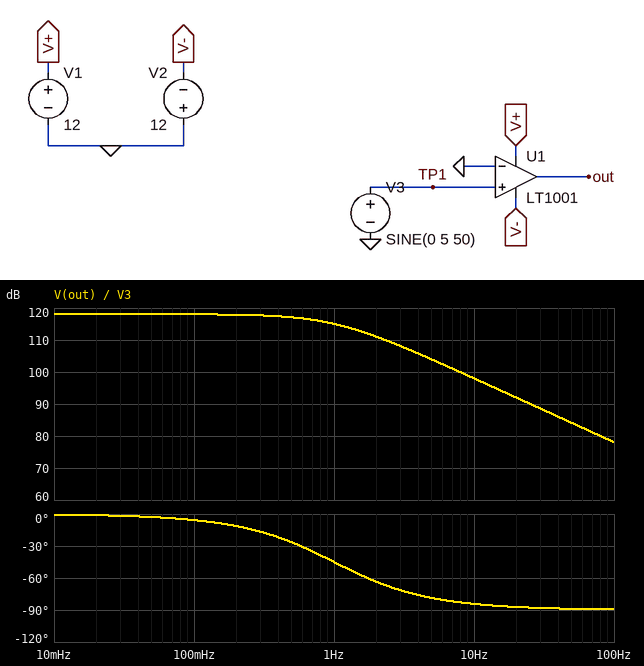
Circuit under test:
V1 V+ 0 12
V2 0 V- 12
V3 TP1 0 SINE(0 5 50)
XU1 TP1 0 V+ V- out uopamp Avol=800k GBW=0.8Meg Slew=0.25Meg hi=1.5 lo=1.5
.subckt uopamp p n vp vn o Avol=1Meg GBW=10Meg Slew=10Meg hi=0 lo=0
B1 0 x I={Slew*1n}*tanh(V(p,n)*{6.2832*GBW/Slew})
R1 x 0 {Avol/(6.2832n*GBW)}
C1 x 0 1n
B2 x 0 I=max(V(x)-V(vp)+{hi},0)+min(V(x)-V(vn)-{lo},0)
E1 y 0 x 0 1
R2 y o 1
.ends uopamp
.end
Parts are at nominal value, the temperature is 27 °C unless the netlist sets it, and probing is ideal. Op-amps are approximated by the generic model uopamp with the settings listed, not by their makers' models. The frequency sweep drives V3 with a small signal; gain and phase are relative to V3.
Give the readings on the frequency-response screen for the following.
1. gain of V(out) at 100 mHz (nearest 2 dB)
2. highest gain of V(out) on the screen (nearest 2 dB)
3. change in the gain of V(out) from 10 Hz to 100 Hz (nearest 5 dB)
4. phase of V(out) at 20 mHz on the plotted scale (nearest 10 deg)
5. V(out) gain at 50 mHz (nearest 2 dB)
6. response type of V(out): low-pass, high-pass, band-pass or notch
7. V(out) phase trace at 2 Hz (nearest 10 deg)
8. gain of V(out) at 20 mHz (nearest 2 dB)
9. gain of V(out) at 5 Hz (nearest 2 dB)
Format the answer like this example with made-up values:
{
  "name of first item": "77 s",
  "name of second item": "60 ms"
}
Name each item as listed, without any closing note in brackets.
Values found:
{
  "gain of V(out) at 100 mHz": "118 dB",
  "highest gain of V(out) on the screen": "118 dB",
  "change in the gain of V(out) from 10 Hz to 100 Hz": "-20 dB",
  "phase of V(out) at 20 mHz on the plotted scale": "0 deg",
  "V(out) gain at 50 mHz": "118 dB",
  "response type of V(out): low-pass, high-pass, band-pass or notch": "low-pass",
  "V(out) phase trace at 2 Hz": "-60 deg",
  "gain of V(out) at 20 mHz": "118 dB",
  "gain of V(out) at 5 Hz": "104 dB"
}
